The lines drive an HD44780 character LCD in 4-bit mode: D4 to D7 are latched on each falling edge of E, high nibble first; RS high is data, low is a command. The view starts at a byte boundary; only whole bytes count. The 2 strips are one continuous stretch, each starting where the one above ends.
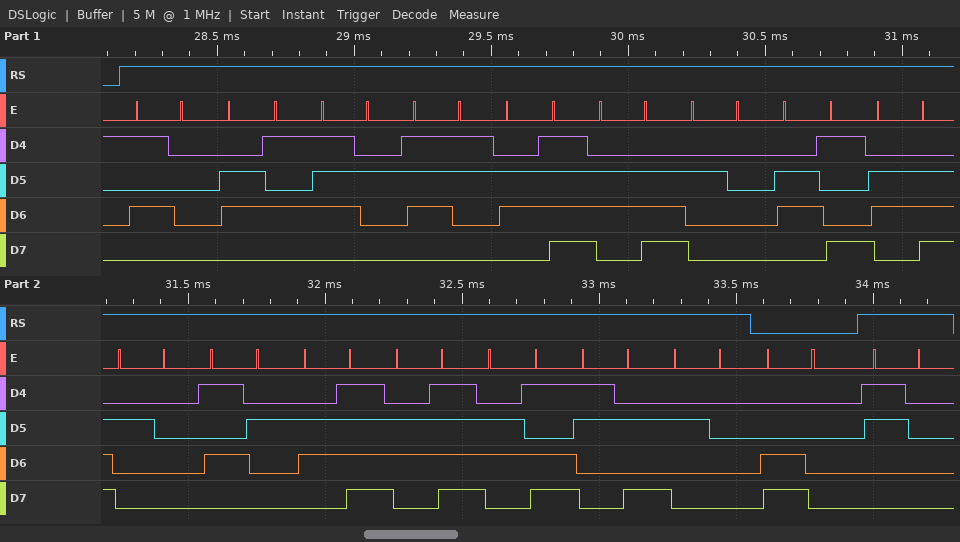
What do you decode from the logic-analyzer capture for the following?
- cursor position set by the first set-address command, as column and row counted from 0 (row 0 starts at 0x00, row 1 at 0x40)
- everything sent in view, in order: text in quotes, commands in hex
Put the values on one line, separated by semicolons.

column 0, row 1; "Person in Room: " 0xC0 "0"
